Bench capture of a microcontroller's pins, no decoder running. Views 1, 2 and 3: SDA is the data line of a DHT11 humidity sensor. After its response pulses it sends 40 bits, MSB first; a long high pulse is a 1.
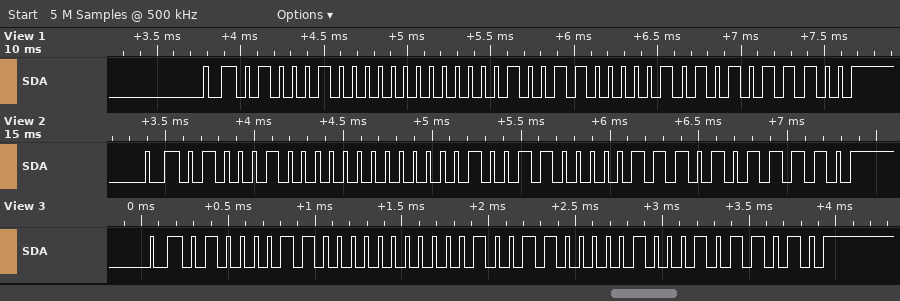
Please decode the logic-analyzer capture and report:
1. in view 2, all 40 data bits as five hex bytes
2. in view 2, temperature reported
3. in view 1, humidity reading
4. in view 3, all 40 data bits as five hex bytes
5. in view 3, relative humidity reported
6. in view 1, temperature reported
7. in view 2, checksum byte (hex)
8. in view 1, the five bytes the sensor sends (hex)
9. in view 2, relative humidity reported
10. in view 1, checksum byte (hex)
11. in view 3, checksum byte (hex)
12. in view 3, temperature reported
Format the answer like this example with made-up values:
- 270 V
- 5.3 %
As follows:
- 44 00 13 07 5E
- 19.7 °C
- 68 %
- 43 00 13 04 5A
- 67 %
- 19.5 °C
- 0x5E
- 44 00 13 05 5C
- 68 %
- 0x5C
- 0x5A
- 19.4 °C
